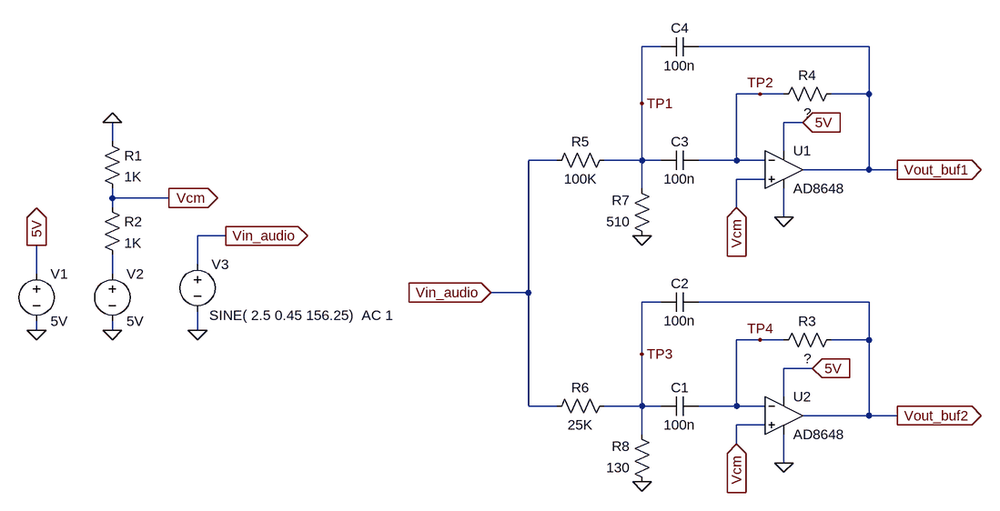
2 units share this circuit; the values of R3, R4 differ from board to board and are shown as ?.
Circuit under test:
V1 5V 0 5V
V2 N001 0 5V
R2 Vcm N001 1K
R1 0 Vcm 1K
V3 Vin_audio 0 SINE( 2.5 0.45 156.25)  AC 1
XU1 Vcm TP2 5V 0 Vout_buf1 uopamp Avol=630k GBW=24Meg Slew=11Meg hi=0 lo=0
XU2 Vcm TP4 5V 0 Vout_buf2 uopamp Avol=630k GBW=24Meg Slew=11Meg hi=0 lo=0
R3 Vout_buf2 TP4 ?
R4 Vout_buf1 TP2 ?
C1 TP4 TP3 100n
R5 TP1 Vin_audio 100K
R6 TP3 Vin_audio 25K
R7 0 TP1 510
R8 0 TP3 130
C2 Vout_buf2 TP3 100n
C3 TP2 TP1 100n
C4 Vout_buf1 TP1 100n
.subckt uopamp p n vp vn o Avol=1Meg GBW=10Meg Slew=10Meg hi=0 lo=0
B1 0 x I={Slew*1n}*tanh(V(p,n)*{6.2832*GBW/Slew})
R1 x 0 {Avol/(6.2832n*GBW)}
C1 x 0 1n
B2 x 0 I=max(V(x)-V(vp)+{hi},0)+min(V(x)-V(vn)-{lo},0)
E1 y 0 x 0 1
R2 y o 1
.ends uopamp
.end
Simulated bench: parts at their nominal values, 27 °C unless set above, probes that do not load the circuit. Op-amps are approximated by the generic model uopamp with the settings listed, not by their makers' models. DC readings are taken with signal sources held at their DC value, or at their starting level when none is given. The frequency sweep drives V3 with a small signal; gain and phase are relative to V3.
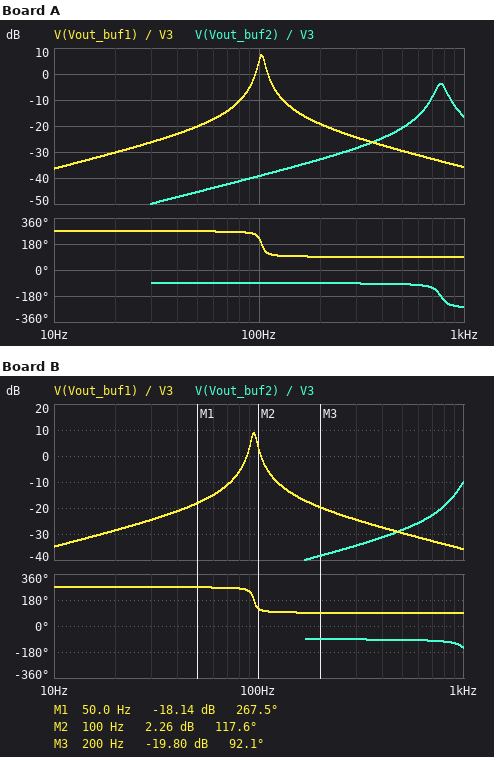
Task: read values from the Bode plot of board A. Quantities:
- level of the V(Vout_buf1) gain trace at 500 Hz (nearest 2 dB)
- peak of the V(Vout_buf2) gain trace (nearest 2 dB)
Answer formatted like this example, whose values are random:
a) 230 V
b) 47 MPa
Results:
a) -30 dB
b) -4 dB
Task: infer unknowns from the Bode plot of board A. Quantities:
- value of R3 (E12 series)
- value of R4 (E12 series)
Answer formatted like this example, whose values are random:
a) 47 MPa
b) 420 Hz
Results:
a) 33 kΩ
b) 470 kΩ
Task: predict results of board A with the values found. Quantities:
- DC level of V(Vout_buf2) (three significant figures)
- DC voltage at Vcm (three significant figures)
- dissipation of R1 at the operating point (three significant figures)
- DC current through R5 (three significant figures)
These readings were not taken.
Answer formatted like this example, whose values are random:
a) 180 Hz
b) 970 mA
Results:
a) 2.50 V
b) 2.50 V
c) 6.25 mW
d) 24.9 µA
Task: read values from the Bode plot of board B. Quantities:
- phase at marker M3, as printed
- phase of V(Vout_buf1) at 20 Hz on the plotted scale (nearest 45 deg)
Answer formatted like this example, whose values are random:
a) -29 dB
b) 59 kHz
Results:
a) 92.1 deg
b) 270 deg
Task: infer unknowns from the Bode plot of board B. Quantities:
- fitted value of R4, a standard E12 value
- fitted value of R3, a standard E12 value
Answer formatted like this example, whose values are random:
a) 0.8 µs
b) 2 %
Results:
a) 560 kΩ
b) 18 kΩ
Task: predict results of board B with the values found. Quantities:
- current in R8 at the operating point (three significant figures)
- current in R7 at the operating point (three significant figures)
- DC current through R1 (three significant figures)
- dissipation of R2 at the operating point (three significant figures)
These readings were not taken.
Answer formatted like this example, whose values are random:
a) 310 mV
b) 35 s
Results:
a) 99.5 µA
b) 24.9 µA
c) 2.50 mA
d) 6.25 mW
